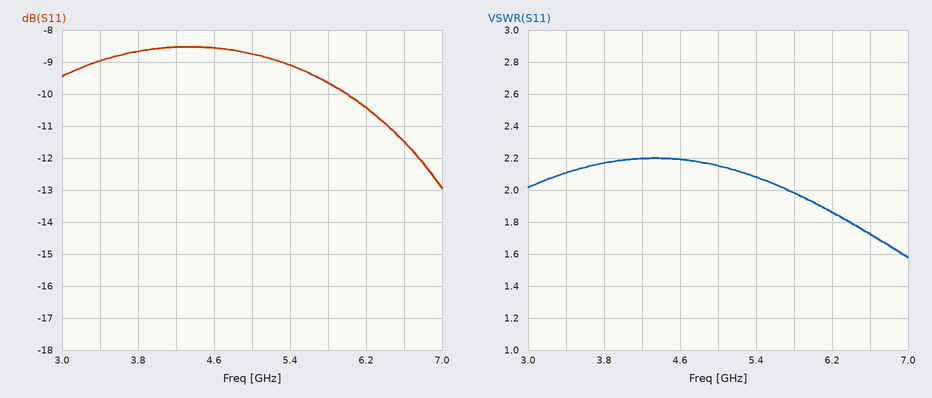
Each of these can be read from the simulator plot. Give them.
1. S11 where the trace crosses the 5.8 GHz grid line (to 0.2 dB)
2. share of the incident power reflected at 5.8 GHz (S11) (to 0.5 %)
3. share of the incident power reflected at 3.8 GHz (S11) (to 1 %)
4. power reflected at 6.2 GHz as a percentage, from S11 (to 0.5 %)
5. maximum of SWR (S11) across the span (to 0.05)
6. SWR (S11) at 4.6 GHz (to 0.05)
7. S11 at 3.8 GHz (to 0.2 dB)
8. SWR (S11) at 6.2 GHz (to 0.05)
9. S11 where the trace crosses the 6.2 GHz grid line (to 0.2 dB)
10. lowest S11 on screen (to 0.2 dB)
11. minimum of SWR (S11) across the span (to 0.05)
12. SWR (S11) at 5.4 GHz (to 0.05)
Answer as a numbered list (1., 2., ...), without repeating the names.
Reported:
1. -9.6 dB
2. 11.0 %
3. 14 %
4. 9.0 %
5. 2.20
6. 2.20
7. -8.6 dB
8. 1.85
9. -10.4 dB
10. -13.0 dB
11. 1.60
12. 2.10
